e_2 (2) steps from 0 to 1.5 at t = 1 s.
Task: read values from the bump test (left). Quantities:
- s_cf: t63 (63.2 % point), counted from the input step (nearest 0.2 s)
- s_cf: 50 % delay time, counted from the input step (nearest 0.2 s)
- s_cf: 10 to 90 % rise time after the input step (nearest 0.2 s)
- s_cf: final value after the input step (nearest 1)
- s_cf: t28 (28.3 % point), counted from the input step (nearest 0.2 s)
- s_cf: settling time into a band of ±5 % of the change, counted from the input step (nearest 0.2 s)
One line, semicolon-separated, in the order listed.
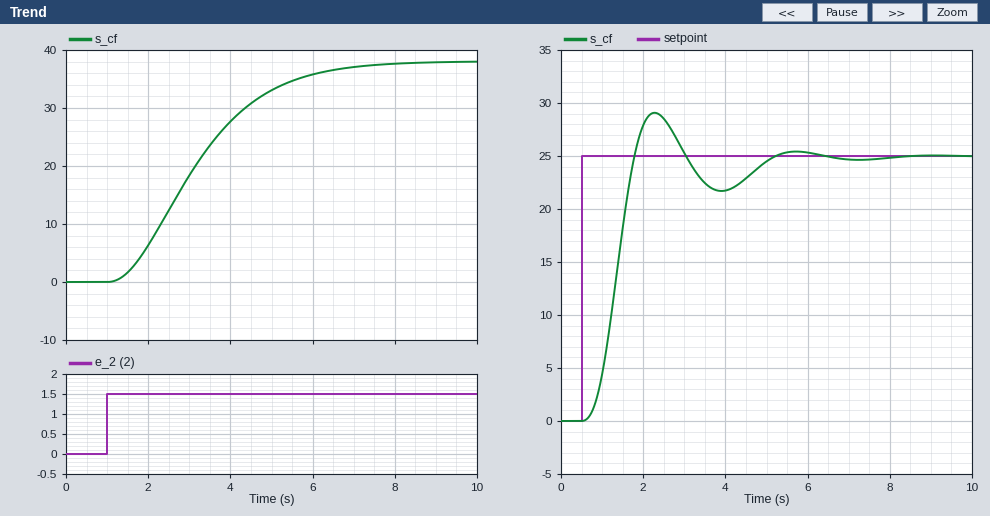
2.6 s; 2.0 s; 3.6 s; 38; 1.4 s; 5.2 s
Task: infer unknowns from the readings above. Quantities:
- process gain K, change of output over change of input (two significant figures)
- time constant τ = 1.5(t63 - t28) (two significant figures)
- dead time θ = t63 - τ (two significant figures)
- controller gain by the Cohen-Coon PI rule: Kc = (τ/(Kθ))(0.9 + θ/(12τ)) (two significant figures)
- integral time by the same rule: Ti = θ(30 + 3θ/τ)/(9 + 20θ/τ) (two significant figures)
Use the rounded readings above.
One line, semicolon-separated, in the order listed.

25; 1.8 s; 0.80 s; 0.084; 1.4 s
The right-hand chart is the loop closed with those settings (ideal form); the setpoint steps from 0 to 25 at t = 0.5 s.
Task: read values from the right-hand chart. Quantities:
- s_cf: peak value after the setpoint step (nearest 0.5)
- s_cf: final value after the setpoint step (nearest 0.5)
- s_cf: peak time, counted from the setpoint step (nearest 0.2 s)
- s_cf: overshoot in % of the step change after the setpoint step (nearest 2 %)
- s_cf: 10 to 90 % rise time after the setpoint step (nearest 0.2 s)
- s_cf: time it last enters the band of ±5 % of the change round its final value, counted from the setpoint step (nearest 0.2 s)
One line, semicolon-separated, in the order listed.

29.0; 25.0; 1.8 s; 16 %; 0.8 s; 4.2 s
